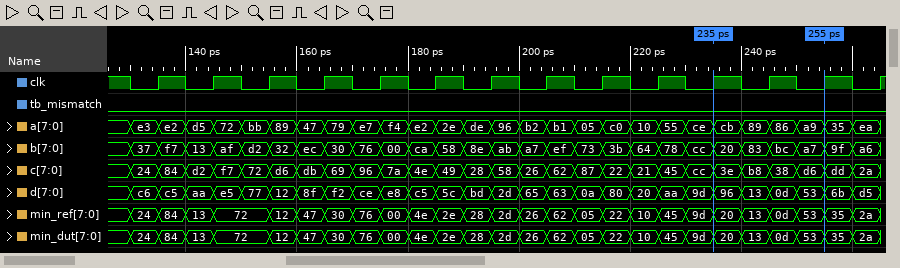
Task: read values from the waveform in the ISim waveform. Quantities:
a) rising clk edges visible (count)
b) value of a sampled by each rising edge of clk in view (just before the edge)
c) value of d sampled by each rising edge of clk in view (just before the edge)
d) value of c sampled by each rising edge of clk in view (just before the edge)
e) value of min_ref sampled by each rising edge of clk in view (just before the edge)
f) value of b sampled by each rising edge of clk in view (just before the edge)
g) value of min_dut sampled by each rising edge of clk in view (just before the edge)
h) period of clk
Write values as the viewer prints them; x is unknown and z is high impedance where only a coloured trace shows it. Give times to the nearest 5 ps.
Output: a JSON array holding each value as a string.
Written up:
["14", "e3, d5, bb, 47, e7, e2, de, b2, 05, 10, ce, 89, a9, ea", "c6, aa, 77, 8f, ce, c5, bd, 65, 0a, 20, 9d, 13, 53, d5", "24, d2, 72, db, 96, 4e, 28, 26, 87, 21, cc, b8, d6, 2a", "24, 13, 72, 47, 76, 4e, 28, 26, 05, 10, 9d, 13, 53, 2a", "37, 13, d2, ec, 76, ca, 8e, a7, 73, 64, cc, 83, a7, a6", "24, 13, 72, 47, 76, 4e, 28, 26, 05, 10, 9d, 13, 53, 2a", "10 ps"]
